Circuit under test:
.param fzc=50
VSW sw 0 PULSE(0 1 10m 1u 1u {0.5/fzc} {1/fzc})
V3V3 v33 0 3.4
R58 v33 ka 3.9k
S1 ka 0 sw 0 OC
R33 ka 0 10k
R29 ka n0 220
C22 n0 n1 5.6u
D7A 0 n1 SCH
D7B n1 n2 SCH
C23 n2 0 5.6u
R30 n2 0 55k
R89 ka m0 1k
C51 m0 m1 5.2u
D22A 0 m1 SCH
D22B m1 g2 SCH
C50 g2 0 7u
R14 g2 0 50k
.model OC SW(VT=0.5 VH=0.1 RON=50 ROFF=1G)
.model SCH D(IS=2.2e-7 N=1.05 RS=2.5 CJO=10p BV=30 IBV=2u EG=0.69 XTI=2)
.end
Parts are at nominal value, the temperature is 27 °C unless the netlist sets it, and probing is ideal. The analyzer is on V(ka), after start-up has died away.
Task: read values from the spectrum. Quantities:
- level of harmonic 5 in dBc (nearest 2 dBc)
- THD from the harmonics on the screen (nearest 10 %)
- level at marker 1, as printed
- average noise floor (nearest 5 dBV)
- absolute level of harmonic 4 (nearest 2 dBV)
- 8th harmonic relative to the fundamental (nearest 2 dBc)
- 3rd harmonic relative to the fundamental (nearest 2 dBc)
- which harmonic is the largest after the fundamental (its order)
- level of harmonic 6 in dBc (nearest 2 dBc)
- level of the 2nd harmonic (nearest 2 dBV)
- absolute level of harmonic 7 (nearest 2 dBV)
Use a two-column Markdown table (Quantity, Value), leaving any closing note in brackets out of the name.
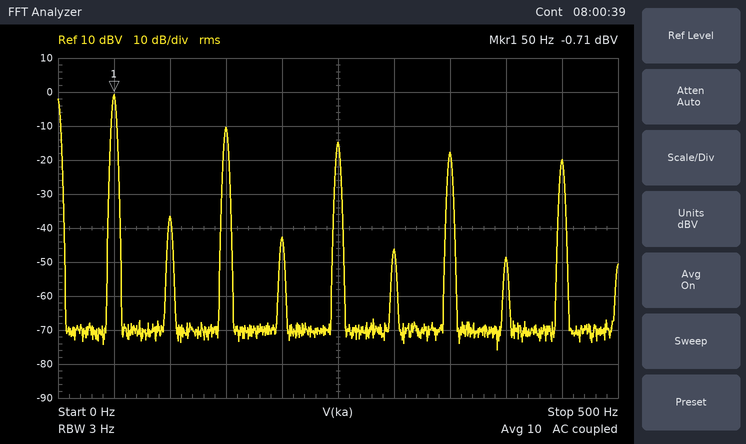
| Quantity | Value |
|---|---|
| level of harmonic 5 in dBc | -14 dBc |
| THD from the harmonics on the screen | 40 % |
| level at marker 1, as printed | -0.71 dBV |
| average noise floor | -70 dBV |
| absolute level of harmonic 4 | -42 dBV |
| 8th harmonic relative to the fundamental | -48 dBc |
| 3rd harmonic relative to the fundamental | -10 dBc |
| which harmonic is the largest after the fundamental | 3 |
| level of harmonic 6 in dBc | -46 dBc |
| level of the 2nd harmonic | -36 dBV |
| absolute level of harmonic 7 | -18 dBV |
